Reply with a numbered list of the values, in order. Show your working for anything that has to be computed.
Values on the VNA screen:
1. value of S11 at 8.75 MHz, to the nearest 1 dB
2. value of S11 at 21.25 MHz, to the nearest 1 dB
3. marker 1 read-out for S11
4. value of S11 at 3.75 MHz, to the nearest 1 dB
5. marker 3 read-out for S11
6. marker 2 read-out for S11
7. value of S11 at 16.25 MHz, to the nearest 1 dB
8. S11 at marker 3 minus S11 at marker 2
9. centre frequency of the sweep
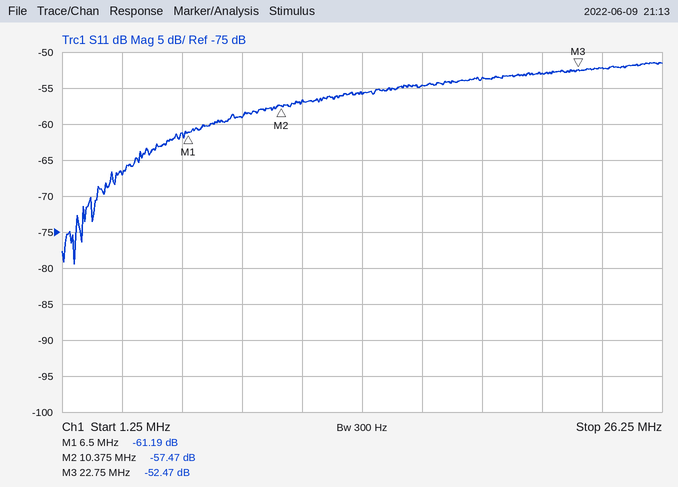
1. -59 dB
2. -53 dB
3. -61.19 dB
4. -67 dB
5. -52.47 dB
6. -57.47 dB
7. -55 dB
8. -52.47 − (-57.47) = 5.00 dB
9. 13.75 MHz
